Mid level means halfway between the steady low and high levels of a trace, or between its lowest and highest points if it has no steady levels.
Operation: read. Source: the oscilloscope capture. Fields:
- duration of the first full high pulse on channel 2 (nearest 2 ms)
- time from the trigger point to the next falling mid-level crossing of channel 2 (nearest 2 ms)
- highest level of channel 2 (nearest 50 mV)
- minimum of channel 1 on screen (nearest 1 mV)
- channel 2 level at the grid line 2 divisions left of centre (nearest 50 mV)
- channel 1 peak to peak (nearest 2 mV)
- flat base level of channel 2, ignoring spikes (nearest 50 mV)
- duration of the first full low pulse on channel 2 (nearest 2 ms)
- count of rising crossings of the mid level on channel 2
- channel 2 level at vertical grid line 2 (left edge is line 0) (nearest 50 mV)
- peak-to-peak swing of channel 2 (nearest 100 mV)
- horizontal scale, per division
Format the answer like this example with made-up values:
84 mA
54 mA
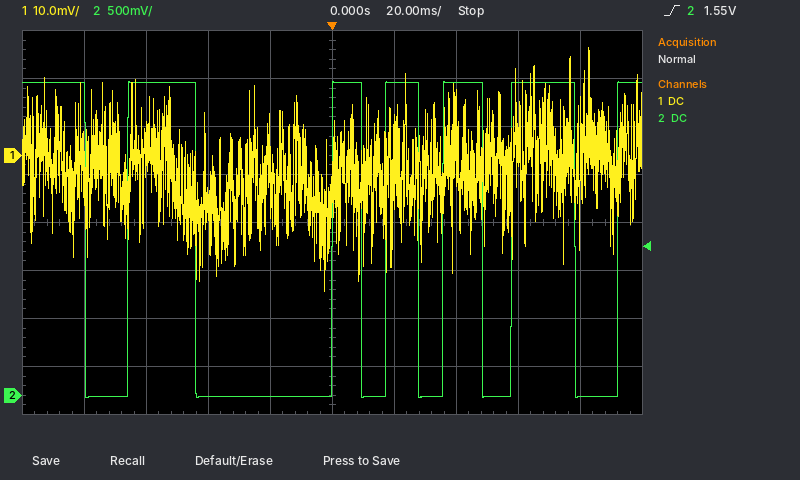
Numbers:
22 ms
10 ms
3.25 V
-28 mV
0 mV
50 mV
0 mV
14 ms
6
3.25 V
3.30 V
20 ms
